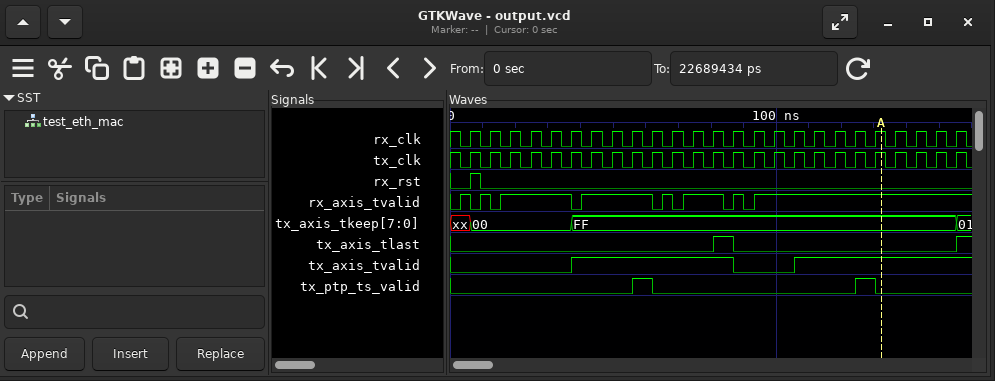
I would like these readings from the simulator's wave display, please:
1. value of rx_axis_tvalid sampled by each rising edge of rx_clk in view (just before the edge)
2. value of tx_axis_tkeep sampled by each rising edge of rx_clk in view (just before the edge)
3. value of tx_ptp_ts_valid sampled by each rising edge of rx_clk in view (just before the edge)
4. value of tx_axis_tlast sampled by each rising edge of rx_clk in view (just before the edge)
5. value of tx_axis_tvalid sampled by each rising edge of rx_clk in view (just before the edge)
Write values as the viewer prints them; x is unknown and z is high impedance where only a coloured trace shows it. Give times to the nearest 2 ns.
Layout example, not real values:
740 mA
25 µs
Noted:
1 1 1 1 1 1 1 1 1 1 1 1 1 0 0 1 1 1 1 1 1 1 1 1 1
xx, 00, 00, 00, 00, 00, FF, FF, FF, FF, FF, FF, FF, FF, FF, FF, FF, FF, FF, FF, FF, FF, FF, FF, FF
0 0 0 0 0 0 0 0 0 1 0 0 0 0 0 0 0 0 0 0 1 0 0 0 0
0 0 0 0 0 0 0 0 0 0 0 0 0 1 0 0 0 0 0 0 0 0 0 0 0
0 0 0 0 0 0 1 1 1 1 1 1 1 1 0 0 0 1 1 1 1 1 1 1 1
